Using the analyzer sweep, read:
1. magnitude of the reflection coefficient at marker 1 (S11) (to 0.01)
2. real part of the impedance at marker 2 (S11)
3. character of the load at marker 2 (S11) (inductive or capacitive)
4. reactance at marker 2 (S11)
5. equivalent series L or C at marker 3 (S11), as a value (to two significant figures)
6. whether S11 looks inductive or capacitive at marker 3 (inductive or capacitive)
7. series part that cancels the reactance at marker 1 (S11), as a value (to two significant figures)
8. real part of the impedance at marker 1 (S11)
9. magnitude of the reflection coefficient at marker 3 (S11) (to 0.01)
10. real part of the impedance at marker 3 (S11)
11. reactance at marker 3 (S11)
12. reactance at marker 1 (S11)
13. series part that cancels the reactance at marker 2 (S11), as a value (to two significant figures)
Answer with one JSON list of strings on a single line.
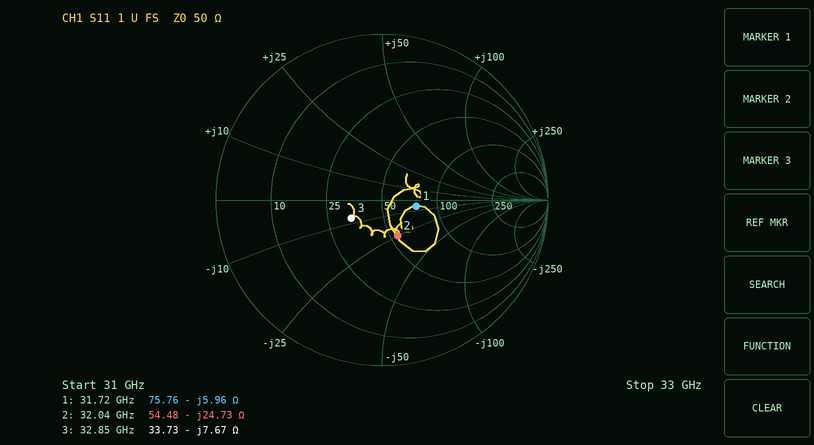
["0.21", "54.48 Ω", "capacitive", "-24.73 Ω", "630 fF", "capacitive", "30 pH", "75.76 Ω", "0.21", "33.73 Ω", "-7.67 Ω", "-5.96 Ω", "120 pH"]
